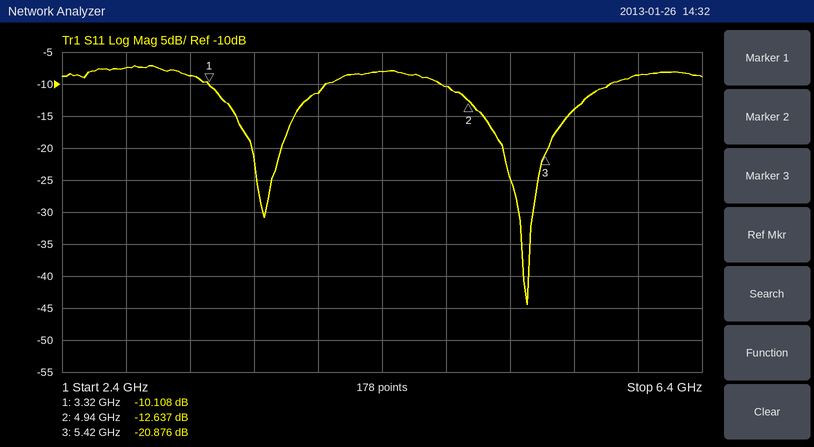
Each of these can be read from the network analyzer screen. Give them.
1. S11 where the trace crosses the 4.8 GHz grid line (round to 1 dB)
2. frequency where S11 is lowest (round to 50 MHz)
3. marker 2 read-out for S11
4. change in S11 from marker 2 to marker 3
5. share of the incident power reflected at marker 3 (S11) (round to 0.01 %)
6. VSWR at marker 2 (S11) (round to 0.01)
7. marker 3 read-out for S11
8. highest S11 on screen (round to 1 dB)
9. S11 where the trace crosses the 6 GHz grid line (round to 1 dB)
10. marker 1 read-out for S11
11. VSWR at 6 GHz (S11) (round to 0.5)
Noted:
-10 dB
5.30 GHz
-12.637 dB
-8.239 dB
0.82 %
1.61
-20.876 dB
-7 dB
-9 dB
-10.108 dB
2.0
